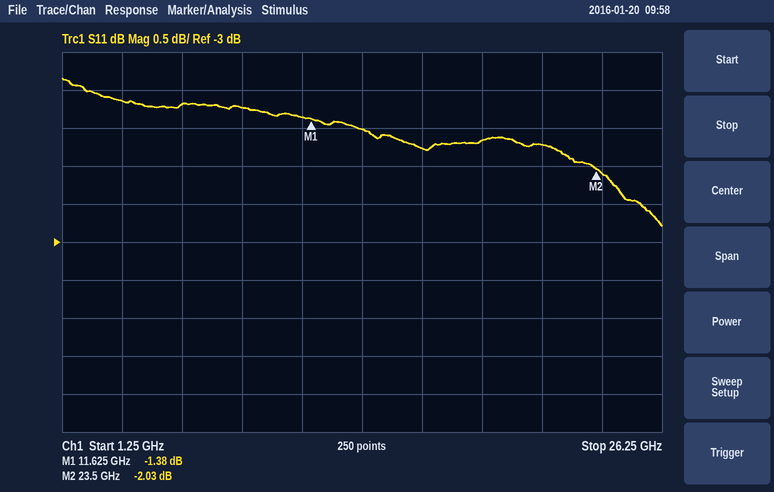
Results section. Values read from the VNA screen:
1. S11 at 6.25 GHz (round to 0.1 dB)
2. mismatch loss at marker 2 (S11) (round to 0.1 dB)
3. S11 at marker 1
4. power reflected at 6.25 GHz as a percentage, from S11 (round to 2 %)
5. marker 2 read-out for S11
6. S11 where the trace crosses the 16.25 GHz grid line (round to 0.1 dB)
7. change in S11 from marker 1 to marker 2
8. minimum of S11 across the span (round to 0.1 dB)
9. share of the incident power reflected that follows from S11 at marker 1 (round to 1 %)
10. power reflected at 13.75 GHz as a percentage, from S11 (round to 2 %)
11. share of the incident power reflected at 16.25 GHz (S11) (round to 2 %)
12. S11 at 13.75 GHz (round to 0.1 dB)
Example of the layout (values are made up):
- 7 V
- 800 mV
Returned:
- -1.2 dB
- 4.3 dB
- -1.38 dB
- 76 %
- -2.03 dB
- -1.8 dB
- -0.65 dB
- -2.8 dB
- 73 %
- 70 %
- 66 %
- -1.5 dB
